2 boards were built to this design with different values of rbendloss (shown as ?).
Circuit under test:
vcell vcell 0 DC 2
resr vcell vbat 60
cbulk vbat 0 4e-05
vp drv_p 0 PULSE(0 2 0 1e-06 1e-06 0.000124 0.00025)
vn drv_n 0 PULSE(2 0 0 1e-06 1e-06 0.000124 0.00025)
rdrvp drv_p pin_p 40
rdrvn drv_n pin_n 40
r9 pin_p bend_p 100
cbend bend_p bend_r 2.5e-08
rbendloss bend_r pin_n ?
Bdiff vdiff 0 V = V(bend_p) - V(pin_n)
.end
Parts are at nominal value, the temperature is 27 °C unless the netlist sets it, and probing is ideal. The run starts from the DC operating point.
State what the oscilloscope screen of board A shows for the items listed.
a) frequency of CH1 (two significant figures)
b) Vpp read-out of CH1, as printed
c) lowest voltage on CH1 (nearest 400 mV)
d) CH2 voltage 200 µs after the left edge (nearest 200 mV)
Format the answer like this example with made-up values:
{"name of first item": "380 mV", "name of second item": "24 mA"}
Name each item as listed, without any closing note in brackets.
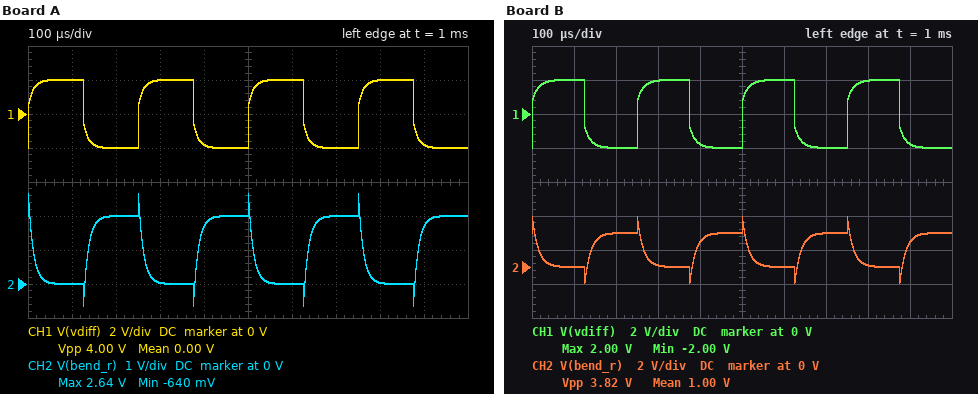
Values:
{"frequency of CH1": "4.0 kHz", "Vpp read-out of CH1, as printed": "4.00 V", "lowest voltage on CH1": "-2.0 V", "CH2 voltage 200 µs after the left edge": "2.0 V"}
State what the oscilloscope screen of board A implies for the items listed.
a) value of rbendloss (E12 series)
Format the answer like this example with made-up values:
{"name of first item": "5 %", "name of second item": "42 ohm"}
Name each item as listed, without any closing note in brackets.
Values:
{"value of rbendloss": "270 Ω"}
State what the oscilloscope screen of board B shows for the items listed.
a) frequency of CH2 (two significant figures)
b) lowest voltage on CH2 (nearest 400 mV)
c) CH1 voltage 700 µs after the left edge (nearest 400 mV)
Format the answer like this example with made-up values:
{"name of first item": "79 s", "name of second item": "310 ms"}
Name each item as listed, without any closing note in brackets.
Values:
{"frequency of CH2": "4.0 kHz", "lowest voltage on CH2": "-800 mV", "CH1 voltage 700 µs after the left edge": "-2.0 V"}
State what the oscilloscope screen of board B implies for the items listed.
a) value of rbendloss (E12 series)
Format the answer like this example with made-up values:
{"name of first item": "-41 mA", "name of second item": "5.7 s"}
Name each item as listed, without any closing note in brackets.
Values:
{"value of rbendloss": "390 Ω"}
